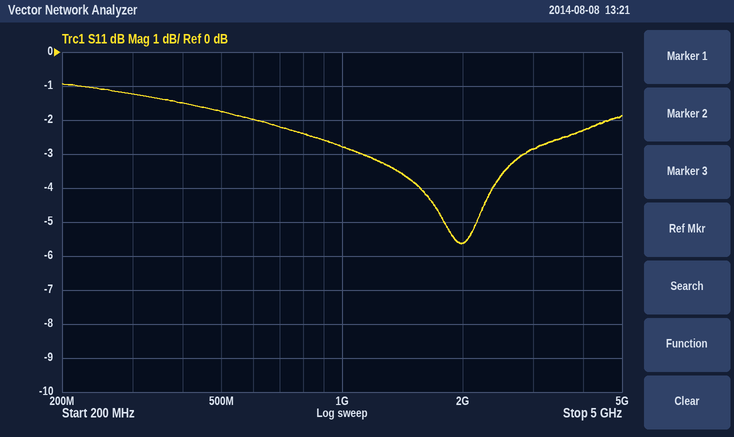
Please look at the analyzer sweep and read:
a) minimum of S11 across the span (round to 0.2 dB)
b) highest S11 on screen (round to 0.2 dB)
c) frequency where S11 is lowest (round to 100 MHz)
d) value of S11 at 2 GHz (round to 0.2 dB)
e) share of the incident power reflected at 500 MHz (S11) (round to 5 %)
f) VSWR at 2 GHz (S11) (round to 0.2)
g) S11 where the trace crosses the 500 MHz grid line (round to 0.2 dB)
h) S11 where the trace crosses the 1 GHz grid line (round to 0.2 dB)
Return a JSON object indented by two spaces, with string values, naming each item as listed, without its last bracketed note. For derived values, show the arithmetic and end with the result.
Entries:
{
  "minimum of S11 across the span": "-5.6 dB",
  "highest S11 on screen": "-1.0 dB",
  "frequency where S11 is lowest": "2.0 GHz",
  "value of S11 at 2 GHz": "-5.6 dB",
  "share of the incident power reflected at 500 MHz (S11)": "10^(-1.8/10) ≈ 66.1 %, so 65 % to the nearest 5 %",
  "VSWR at 2 GHz (S11)": "|Γ| = 10^(-5.6/20) = 0.5248; VSWR = (1 + 0.5248)/(1 − 0.5248) ≈ 3.2",
  "S11 where the trace crosses the 500 MHz grid line": "-1.8 dB",
  "S11 where the trace crosses the 1 GHz grid line": "-2.8 dB"
}
